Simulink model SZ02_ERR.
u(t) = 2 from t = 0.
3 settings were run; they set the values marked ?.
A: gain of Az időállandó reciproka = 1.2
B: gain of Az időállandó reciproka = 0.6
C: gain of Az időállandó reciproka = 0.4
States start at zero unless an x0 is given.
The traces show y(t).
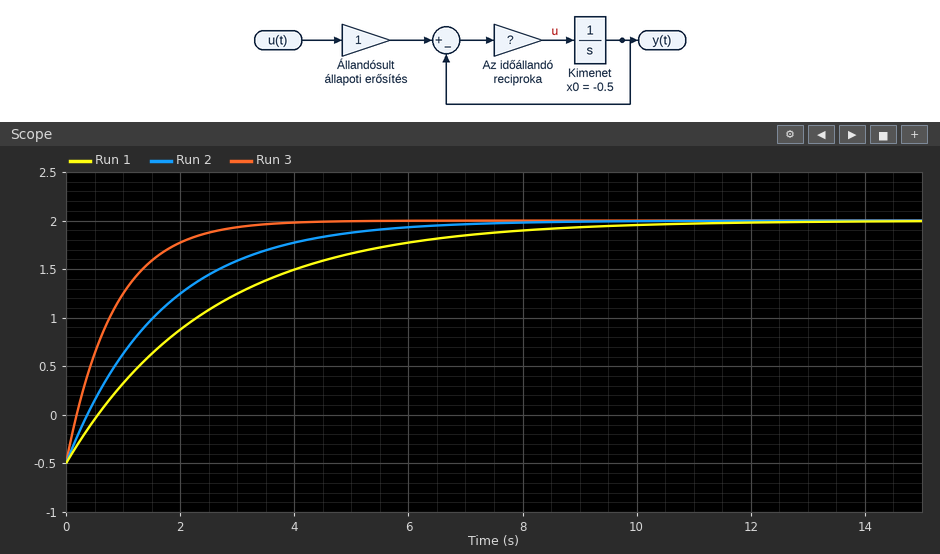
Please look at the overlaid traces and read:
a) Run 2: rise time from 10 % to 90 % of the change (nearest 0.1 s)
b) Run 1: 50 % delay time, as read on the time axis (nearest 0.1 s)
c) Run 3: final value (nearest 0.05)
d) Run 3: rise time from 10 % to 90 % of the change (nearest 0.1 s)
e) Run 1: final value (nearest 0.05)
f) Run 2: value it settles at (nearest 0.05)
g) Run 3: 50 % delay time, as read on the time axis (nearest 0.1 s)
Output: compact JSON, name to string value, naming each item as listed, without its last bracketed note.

{"Run 2: rise time from 10 % to 90 % of the change": "3.7 s", "Run 1: 50 % delay time, as read on the time axis": "1.7 s", "Run 3: final value": "2.00", "Run 3: rise time from 10 % to 90 % of the change": "1.8 s", "Run 1: final value": "2.00", "Run 2: value it settles at": "2.00", "Run 3: 50 % delay time, as read on the time axis": "0.6 s"}
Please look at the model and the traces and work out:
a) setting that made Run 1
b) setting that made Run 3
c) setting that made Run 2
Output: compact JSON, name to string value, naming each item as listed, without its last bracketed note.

{"setting that made Run 1": "C", "setting that made Run 3": "A", "setting that made Run 2": "B"}
